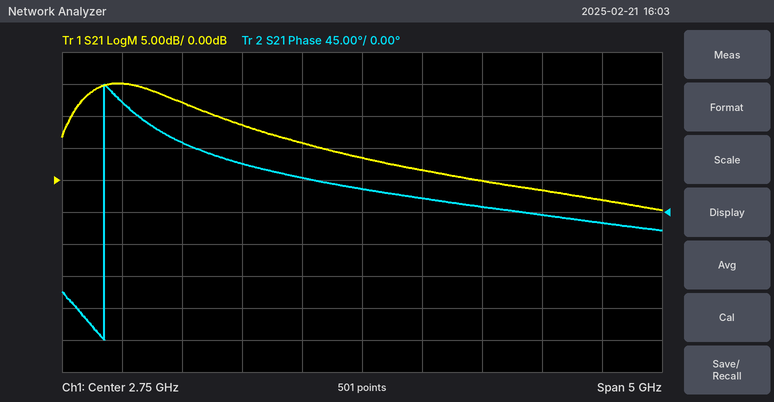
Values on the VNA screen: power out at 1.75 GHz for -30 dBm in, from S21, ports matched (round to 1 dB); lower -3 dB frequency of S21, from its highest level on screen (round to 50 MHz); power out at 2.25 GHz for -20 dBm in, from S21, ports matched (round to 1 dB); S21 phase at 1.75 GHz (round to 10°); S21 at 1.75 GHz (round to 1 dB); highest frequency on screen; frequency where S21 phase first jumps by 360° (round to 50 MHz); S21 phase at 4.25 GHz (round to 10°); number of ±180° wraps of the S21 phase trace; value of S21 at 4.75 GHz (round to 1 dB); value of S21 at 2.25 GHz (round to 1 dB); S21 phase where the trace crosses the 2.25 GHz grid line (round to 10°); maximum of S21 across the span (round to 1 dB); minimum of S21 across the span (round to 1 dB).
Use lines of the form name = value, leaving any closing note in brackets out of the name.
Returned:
power out at 1.75 GHz for -30 dBm in, from S21, ports matched = -21 dBm
lower -3 dB frequency of S21, from its highest level on screen = 400 MHz
power out at 2.25 GHz for -20 dBm in, from S21, ports matched = -14 dBm
S21 phase at 1.75 GHz = 70°
S21 at 1.75 GHz = 9 dB
highest frequency on screen = 5.25 GHz
frequency where S21 phase first jumps by 360° = 600 MHz
S21 phase at 4.25 GHz = 0°
number of ±180° wraps of the S21 phase trace = 1
value of S21 at 4.75 GHz = -3 dB
value of S21 at 2.25 GHz = 6 dB
S21 phase where the trace crosses the 2.25 GHz grid line = 50°
maximum of S21 across the span = 15 dB
minimum of S21 across the span = -5 dB
